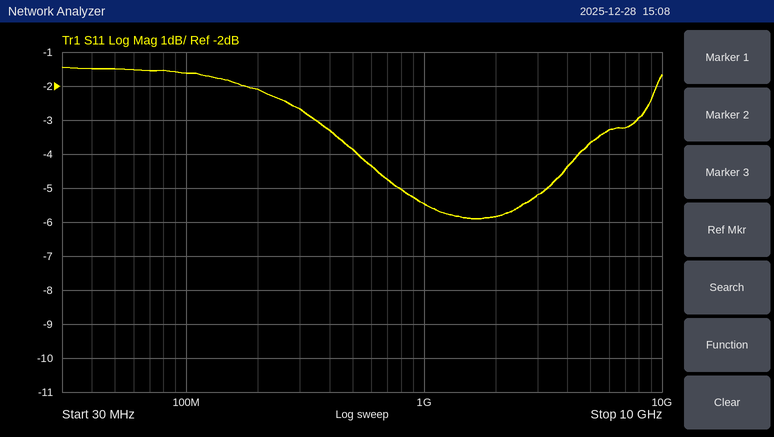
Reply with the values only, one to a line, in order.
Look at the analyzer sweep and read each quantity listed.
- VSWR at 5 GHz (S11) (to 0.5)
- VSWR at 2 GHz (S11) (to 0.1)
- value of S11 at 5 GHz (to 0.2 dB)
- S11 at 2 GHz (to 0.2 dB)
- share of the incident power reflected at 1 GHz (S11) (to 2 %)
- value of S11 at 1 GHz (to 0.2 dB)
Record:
5.0
3.1
-3.6 dB
-5.8 dB
28 %
-5.4 dB
